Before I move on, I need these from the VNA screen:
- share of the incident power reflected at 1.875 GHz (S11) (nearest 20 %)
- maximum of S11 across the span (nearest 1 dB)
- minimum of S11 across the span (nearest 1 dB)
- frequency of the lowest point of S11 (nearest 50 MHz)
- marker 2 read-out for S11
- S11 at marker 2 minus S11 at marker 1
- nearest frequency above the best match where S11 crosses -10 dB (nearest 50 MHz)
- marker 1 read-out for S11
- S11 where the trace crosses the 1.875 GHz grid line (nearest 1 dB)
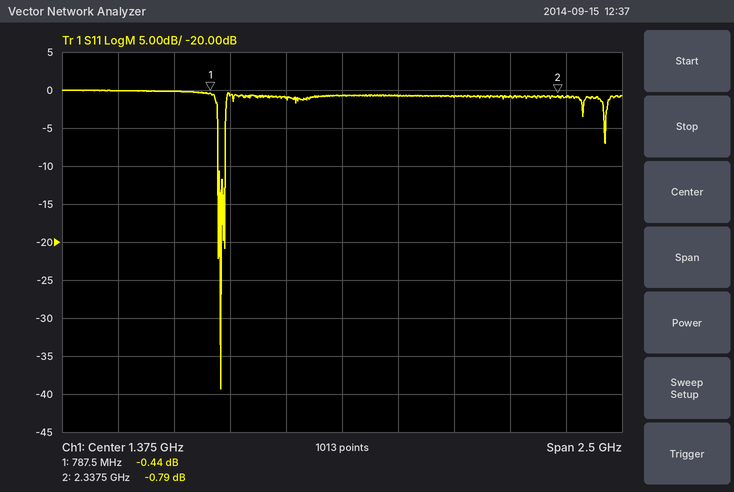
80 %
0 dB
-39 dB
850 MHz
-0.79 dB
-0.35 dB
850 MHz
-0.44 dB
-1 dB
